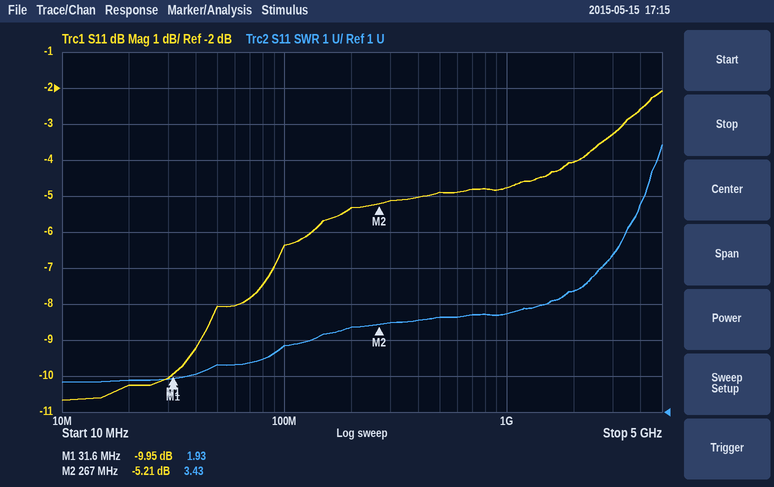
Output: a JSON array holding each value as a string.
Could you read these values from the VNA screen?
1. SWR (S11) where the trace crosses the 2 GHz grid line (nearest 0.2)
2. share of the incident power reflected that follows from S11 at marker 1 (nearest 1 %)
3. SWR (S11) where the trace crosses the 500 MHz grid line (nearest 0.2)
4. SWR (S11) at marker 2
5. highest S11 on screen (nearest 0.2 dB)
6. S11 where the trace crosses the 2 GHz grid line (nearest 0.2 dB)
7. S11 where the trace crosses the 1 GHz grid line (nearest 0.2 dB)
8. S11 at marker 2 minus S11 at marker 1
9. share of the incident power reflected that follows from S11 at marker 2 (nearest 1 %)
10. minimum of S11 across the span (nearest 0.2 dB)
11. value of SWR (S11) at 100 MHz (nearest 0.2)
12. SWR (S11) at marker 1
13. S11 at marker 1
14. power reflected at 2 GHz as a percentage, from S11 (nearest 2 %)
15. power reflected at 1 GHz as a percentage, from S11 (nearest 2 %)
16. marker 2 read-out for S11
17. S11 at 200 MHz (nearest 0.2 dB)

["4.4", "10 %", "3.6", "3.43", "-2.0 dB", "-4.0 dB", "-4.8 dB", "4.74 dB", "30 %", "-10.6 dB", "2.8", "1.93", "-9.95 dB", "40 %", "34 %", "-5.21 dB", "-5.4 dB"]
